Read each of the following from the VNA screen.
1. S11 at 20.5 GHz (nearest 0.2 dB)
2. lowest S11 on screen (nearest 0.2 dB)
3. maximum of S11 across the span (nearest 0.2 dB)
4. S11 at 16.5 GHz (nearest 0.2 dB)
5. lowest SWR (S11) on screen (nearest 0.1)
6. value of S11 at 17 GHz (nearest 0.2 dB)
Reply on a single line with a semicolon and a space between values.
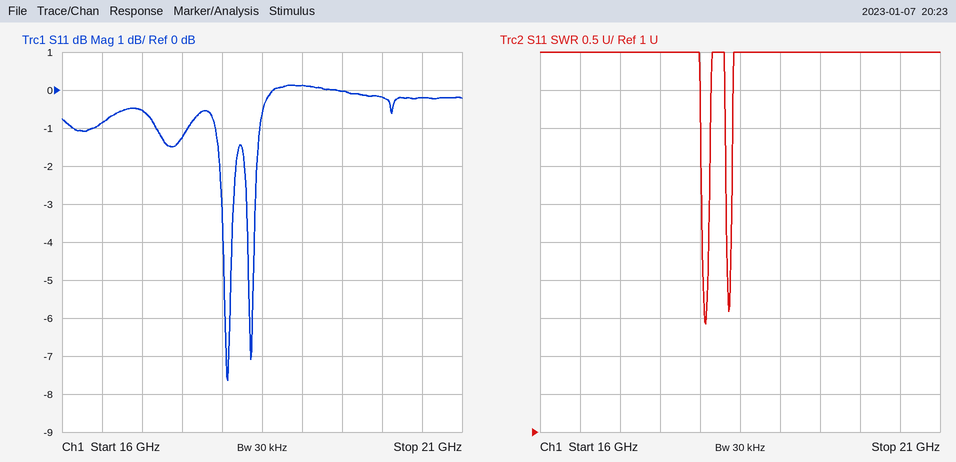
-0.2 dB; -7.6 dB; 0.2 dB; -0.8 dB; 2.4; -0.6 dB
